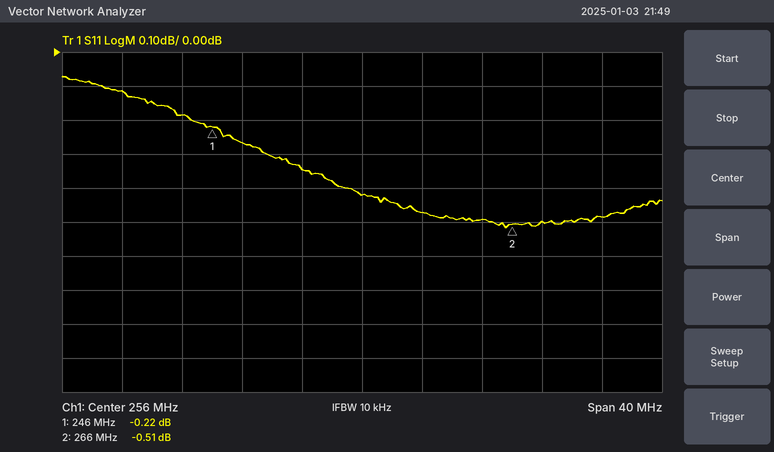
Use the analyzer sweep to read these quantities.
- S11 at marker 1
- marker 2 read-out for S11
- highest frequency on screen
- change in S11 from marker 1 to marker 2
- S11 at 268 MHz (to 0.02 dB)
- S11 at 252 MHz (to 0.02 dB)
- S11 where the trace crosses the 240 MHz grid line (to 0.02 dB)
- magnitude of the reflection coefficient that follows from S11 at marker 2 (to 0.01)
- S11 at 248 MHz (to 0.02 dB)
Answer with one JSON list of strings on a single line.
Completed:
["-0.22 dB", "-0.51 dB", "276 MHz", "-0.29 dB", "-0.50 dB", "-0.34 dB", "-0.12 dB", "0.94", "-0.26 dB"]
